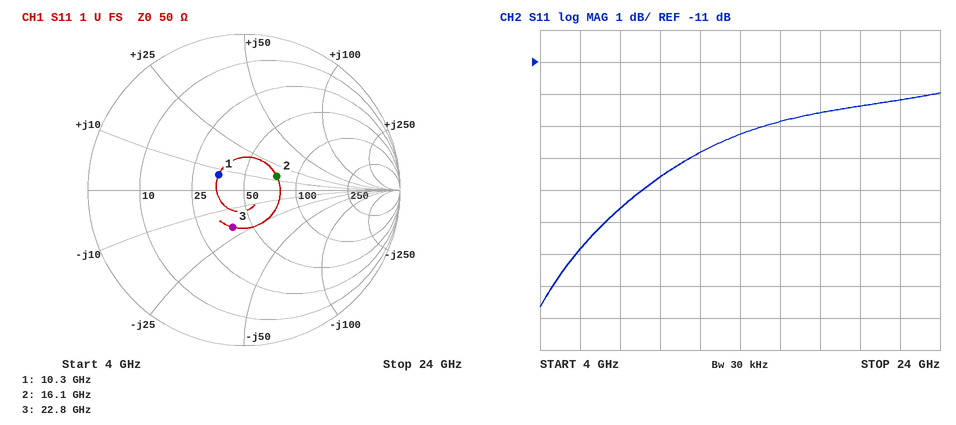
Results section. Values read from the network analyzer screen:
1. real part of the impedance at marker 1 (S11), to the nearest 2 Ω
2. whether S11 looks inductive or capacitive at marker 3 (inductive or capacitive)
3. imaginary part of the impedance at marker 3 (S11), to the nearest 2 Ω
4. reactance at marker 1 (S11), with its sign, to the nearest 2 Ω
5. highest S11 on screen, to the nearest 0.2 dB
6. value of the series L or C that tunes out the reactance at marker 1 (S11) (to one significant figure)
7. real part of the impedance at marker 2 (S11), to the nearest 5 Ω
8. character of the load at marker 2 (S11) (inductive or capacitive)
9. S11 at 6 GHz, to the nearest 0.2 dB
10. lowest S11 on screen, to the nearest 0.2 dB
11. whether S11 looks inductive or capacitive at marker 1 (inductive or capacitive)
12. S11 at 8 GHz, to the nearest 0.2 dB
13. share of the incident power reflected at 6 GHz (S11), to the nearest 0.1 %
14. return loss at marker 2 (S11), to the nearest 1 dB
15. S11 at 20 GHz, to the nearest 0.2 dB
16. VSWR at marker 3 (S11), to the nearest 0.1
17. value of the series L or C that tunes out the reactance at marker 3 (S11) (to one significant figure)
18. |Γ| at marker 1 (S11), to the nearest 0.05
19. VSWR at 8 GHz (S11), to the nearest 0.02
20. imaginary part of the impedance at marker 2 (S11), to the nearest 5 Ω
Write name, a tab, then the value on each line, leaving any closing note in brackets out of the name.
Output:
real part of the impedance at marker 1 (S11), to the nearest 2 Ω	36 Ω
whether S11 looks inductive or capacitive at marker 3	capacitive
imaginary part of the impedance at marker 3 (S11), to the nearest 2 Ω	-20 Ω
reactance at marker 1 (S11), with its sign, to the nearest 2 Ω	+8 Ω
highest S11 on screen, to the nearest 0.2 dB	-12.0 dB
value of the series L or C that tunes out the reactance at marker 1 (S11)	2 pF
real part of the impedance at marker 2 (S11), to the nearest 5 Ω	75 Ω
character of the load at marker 2 (S11)	inductive
S11 at 6 GHz, to the nearest 0.2 dB	-16.8 dB
lowest S11 on screen, to the nearest 0.2 dB	-18.6 dB
whether S11 looks inductive or capacitive at marker 1	inductive
S11 at 8 GHz, to the nearest 0.2 dB	-15.6 dB
share of the incident power reflected at 6 GHz (S11), to the nearest 0.1 %	2.1 %
return loss at marker 2 (S11), to the nearest 1 dB	13 dB
S11 at 20 GHz, to the nearest 0.2 dB	-12.4 dB
VSWR at marker 3 (S11), to the nearest 0.1	1.7
value of the series L or C that tunes out the reactance at marker 3 (S11)	100 pH
|Γ| at marker 1 (S11), to the nearest 0.05	0.20
VSWR at 8 GHz (S11), to the nearest 0.02	1.40
imaginary part of the impedance at marker 2 (S11), to the nearest 5 Ω	+15 Ω
